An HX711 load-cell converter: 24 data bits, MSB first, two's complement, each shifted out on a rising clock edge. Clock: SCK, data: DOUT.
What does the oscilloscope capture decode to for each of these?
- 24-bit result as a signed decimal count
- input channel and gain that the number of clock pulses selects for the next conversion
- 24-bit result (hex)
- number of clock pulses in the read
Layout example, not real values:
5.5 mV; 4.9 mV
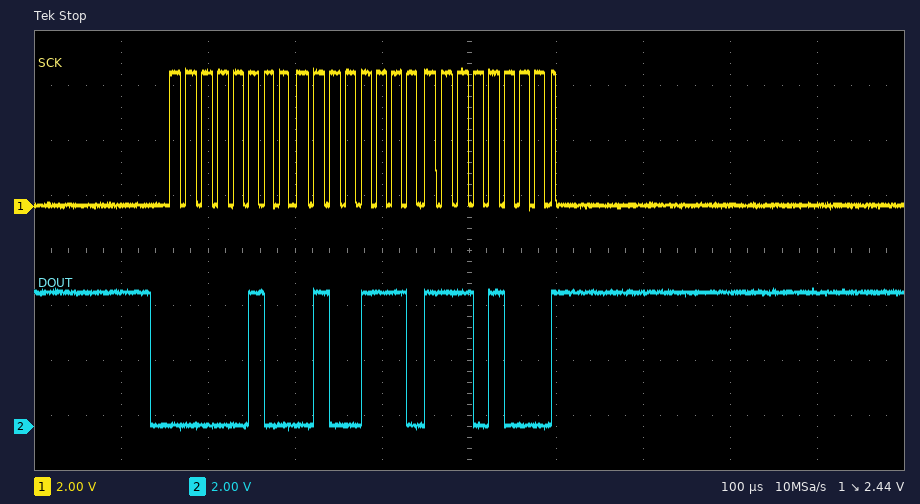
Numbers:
282344; channel A, gain 128; 0x044EE8; 25
